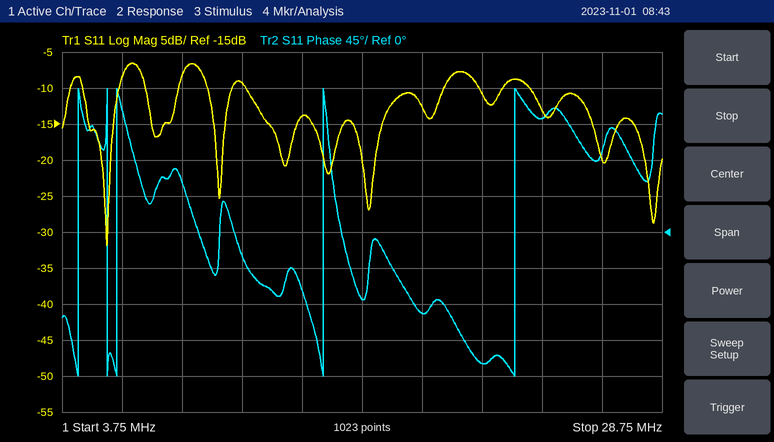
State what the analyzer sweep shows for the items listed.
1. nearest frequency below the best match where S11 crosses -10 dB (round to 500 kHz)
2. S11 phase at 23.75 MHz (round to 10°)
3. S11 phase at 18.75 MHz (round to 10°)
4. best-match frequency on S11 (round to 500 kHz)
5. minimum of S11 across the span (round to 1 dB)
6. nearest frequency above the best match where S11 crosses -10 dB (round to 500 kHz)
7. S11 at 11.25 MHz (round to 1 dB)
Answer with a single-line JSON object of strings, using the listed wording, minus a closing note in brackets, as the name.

{"nearest frequency below the best match where S11 crosses -10 dB": "4.5 MHz", "S11 phase at 23.75 MHz": "140°", "S11 phase at 18.75 MHz": "-100°", "best-match frequency on S11": "5.5 MHz", "minimum of S11 across the span": "-32 dB", "nearest frequency above the best match where S11 crosses -10 dB": "6.0 MHz", "S11 at 11.25 MHz": "-9 dB"}
